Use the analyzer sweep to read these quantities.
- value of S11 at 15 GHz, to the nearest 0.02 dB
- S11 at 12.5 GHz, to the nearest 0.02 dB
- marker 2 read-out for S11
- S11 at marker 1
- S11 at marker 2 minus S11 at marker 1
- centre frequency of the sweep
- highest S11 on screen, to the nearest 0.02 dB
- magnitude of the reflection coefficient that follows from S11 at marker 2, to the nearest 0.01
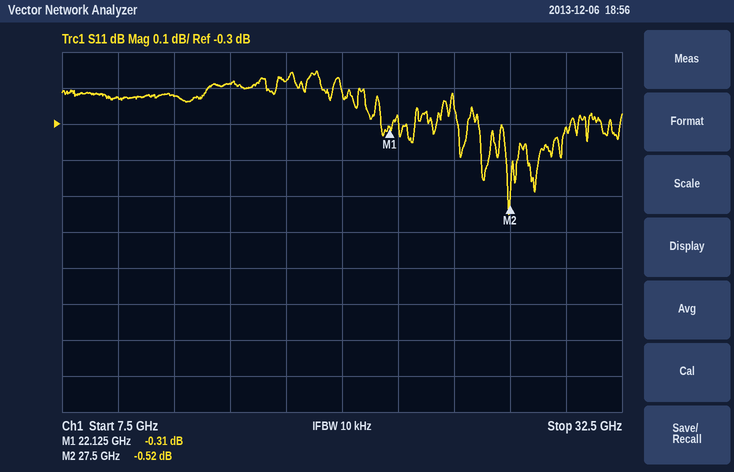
-0.18 dB
-0.22 dB
-0.52 dB
-0.31 dB
-0.21 dB
20 GHz
-0.16 dB
0.94
